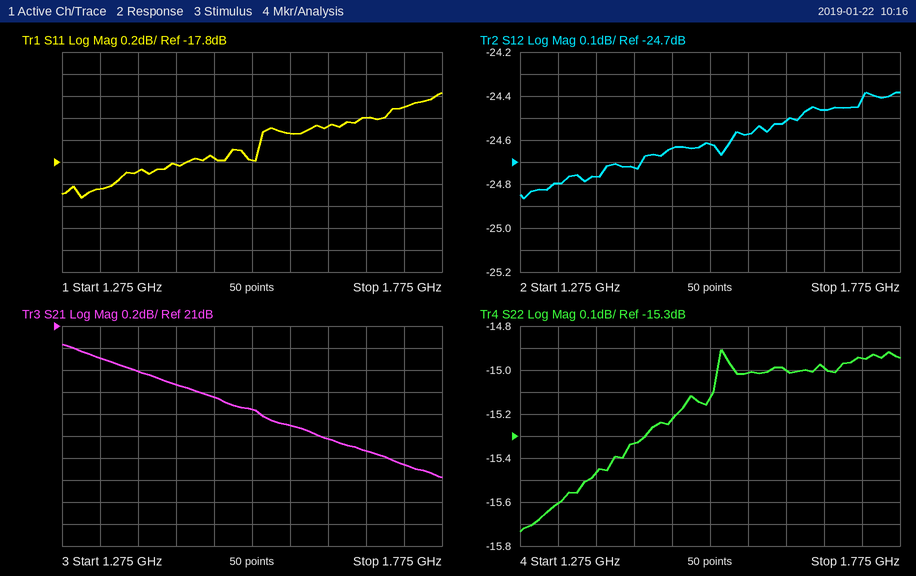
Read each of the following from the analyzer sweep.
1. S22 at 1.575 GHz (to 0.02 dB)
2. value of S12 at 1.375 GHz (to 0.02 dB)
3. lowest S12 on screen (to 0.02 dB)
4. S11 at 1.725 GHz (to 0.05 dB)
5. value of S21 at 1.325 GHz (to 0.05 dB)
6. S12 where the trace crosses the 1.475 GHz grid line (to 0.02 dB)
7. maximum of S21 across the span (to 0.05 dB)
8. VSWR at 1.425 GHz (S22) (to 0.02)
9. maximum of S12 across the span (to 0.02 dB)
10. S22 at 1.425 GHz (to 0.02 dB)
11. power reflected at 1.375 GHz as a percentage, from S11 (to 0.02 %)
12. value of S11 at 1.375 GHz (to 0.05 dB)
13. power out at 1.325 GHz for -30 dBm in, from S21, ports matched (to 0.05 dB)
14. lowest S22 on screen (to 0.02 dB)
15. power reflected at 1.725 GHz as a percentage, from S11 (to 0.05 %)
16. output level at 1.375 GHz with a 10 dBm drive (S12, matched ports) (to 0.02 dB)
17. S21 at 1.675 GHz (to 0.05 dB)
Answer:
-15.02 dB
-24.76 dB
-24.86 dB
-17.30 dB
20.70 dB
-24.64 dB
20.85 dB
1.42
-24.38 dB
-15.34 dB
1.62 %
-17.90 dB
-9.30 dBm
-15.74 dB
1.85 %
-14.76 dBm
19.85 dB
